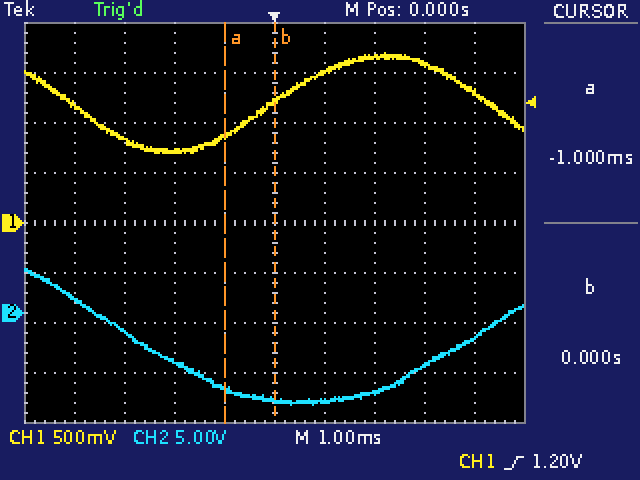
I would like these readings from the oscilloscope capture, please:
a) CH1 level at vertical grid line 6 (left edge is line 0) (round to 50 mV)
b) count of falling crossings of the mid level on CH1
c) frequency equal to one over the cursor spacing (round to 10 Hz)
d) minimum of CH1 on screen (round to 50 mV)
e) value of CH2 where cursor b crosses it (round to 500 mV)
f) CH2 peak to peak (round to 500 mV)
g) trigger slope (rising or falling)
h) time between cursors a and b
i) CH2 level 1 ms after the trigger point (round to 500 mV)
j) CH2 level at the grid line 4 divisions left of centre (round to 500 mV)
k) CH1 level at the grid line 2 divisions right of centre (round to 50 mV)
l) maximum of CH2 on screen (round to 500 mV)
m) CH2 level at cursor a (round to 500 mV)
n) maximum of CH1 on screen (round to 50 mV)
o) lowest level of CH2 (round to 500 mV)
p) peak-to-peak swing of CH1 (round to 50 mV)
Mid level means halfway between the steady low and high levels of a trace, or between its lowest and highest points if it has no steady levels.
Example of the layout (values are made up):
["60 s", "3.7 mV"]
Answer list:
["1.50 V", "2", "1.00 kHz", "700 mV", "-8.5 V", "13.5 V", "rising", "1.0 ms", "-9.0 V", "1.5 V", "1.65 V", "4.5 V", "-7.5 V", "1.70 V", "-9.0 V", "1.00 V"]
